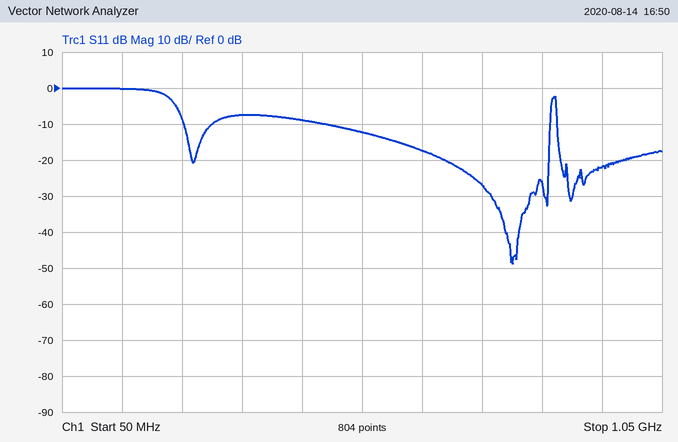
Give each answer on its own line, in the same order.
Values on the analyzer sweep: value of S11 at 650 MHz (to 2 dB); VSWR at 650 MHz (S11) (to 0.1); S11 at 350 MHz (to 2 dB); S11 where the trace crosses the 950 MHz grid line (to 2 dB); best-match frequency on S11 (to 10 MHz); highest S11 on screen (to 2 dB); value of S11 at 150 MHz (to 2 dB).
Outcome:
-18 dB
1.3
-8 dB
-22 dB
800 MHz
0 dB
0 dB
